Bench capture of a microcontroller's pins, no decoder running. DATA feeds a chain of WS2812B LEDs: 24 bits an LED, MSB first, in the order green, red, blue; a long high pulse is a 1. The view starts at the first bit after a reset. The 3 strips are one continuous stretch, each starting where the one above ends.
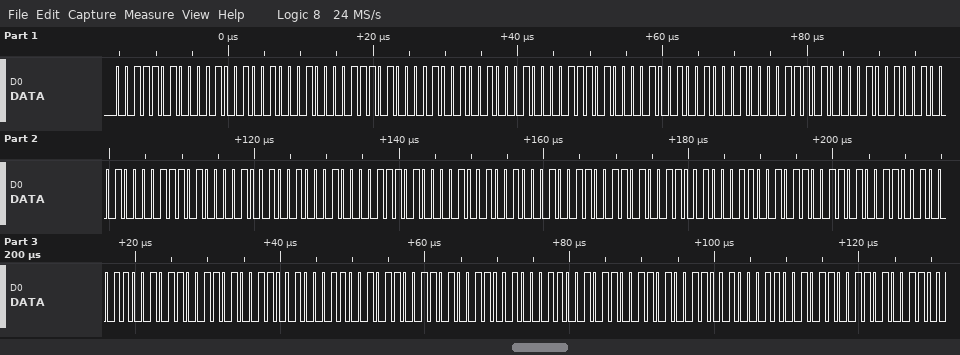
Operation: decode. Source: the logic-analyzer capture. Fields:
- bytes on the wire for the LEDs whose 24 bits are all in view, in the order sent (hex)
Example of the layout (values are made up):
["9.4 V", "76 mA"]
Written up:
["3A 12 44 3A 12 44 3A 12 44 3A 12 44 3A 12 44 3A 12 44 CD 32 32 CD 32 32 CD 32 32 CD 32 32 CD 32 32"]
